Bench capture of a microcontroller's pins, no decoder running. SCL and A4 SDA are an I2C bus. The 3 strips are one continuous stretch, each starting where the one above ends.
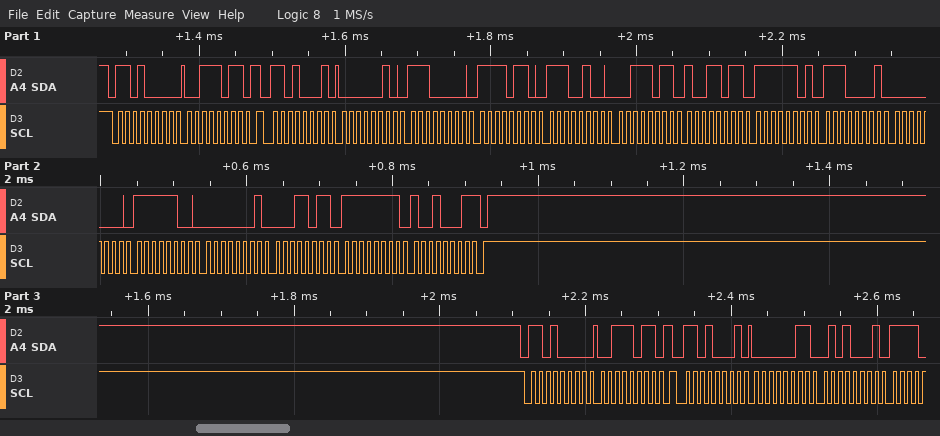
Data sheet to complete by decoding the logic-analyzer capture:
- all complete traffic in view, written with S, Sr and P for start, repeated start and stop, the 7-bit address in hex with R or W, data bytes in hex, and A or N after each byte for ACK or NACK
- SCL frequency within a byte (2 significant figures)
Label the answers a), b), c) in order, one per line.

a) S 68W A 3B A Sr 68R A 02 A E0 A F6 A E4 A 3B A 9B A FD A E1 A 00 A FC A 01 A 1B A FF A 91 N P S 68W A 3B A Sr 68R A 03 A 51 A
b) 100 kHz
